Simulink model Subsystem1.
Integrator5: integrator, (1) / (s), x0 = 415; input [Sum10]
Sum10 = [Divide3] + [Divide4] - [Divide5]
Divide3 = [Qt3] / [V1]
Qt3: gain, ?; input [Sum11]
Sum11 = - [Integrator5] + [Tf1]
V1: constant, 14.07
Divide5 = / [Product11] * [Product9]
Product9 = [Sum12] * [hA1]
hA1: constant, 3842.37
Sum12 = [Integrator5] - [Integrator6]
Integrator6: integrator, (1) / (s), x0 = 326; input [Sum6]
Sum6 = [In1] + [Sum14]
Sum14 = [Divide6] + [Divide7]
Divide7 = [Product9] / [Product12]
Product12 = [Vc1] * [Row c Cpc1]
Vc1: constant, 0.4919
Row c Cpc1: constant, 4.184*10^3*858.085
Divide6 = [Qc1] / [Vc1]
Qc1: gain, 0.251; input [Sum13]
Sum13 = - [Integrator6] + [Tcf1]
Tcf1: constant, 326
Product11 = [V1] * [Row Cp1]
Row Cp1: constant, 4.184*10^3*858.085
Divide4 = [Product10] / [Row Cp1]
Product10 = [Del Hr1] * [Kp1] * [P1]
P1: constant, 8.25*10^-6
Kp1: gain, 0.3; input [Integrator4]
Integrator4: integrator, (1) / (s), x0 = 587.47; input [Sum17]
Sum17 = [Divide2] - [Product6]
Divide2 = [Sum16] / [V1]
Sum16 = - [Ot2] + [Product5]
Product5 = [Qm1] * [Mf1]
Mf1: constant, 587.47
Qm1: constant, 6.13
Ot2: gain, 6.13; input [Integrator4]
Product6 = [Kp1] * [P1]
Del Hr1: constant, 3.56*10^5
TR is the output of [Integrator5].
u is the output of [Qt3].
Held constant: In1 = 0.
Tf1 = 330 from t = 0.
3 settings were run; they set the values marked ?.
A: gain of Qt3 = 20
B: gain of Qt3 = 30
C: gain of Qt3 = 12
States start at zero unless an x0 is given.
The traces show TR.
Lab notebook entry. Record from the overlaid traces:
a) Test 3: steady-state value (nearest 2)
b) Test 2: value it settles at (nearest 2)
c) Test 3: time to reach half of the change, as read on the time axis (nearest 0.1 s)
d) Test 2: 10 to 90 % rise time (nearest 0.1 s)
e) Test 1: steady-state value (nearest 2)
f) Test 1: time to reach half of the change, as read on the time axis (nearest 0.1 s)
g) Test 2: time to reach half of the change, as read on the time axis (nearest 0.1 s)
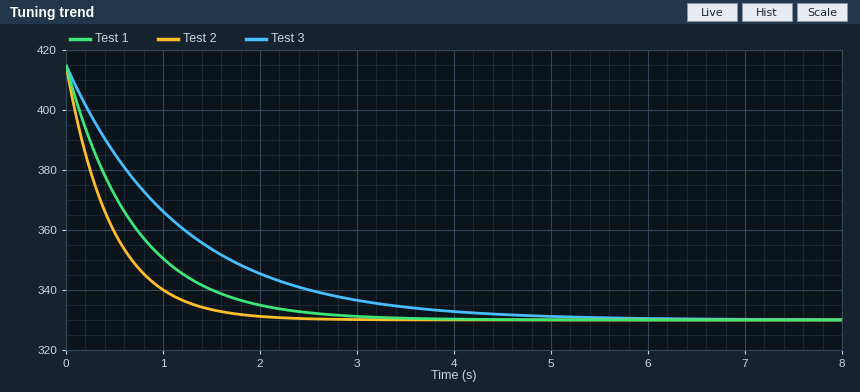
330
330
0.8 s
1.0 s
330
0.5 s
0.3 s
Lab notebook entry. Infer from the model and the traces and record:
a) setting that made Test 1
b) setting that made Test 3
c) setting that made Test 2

A
C
B
